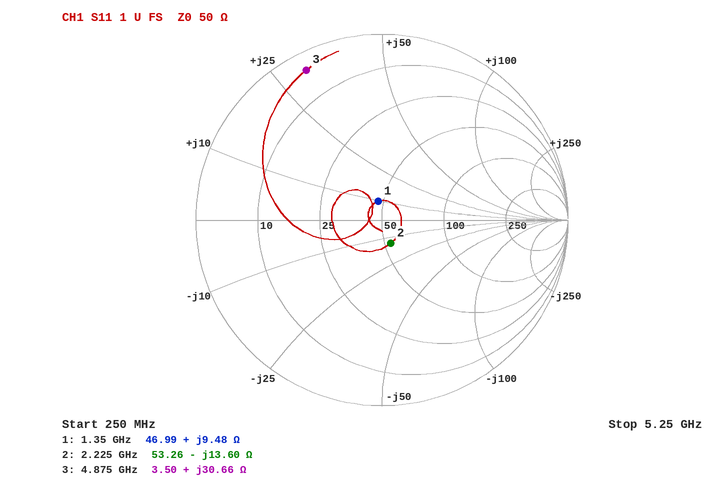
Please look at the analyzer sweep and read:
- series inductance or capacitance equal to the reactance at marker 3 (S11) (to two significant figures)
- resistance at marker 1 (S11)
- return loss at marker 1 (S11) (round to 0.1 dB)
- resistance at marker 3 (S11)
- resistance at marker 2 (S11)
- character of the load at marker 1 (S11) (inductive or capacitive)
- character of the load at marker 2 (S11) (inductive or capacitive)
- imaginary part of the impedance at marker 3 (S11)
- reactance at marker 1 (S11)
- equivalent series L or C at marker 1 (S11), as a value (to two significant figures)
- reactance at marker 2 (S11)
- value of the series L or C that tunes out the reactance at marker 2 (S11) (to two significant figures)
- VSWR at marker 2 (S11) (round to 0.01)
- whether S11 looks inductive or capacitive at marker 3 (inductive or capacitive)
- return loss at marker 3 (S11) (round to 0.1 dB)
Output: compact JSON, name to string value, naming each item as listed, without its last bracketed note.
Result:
{"series inductance or capacitance equal to the reactance at marker 3 (S11)": "1.0 nH", "resistance at marker 1": "46.99 Ω", "return loss at marker 1 (S11)": "19.8 dB", "resistance at marker 3": "3.50 Ω", "resistance at marker 2": "53.26 Ω", "character of the load at marker 1 (S11)": "inductive", "character of the load at marker 2 (S11)": "capacitive", "imaginary part of the impedance at marker 3": "+30.66 Ω", "reactance at marker 1": "+9.48 Ω", "equivalent series L or C at marker 1 (S11), as a value": "1.1 nH", "reactance at marker 2": "-13.60 Ω", "value of the series L or C that tunes out the reactance at marker 2 (S11)": "970 pH", "VSWR at marker 2 (S11)": "1.31", "whether S11 looks inductive or capacitive at marker 3": "inductive", "return loss at marker 3 (S11)": "0.9 dB"}
